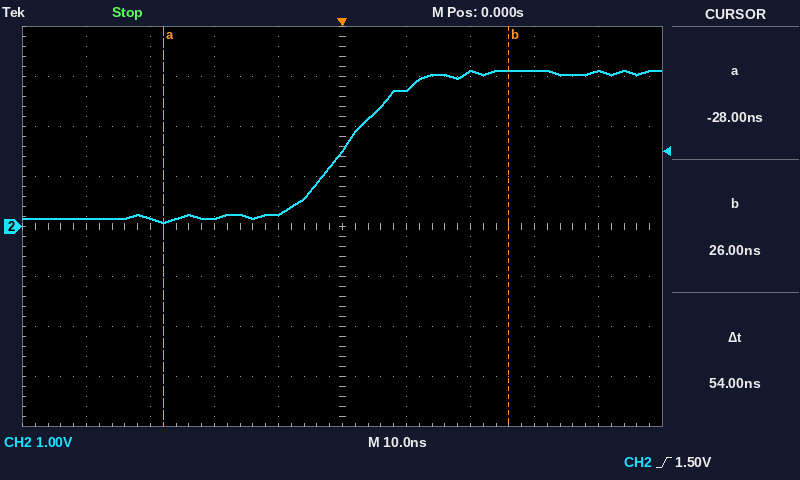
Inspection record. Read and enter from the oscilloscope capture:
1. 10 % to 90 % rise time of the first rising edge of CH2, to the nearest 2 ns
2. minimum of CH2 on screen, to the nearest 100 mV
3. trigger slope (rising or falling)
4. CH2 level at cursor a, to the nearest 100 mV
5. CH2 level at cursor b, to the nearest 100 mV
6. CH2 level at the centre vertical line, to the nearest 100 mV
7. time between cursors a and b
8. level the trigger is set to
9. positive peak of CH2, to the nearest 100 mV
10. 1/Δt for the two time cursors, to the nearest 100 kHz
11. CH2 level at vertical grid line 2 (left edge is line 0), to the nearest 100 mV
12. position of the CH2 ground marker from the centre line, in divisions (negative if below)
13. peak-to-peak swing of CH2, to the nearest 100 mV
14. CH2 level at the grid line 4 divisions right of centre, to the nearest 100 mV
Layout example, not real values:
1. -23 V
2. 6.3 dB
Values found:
1. 18 ns
2. 100 mV
3. rising
4. 100 mV
5. 3.1 V
6. 1.5 V
7. 54 ns
8. 1.50 V
9. 3.1 V
10. 18.5 MHz
11. 200 mV
12. 0.0 div
13. 3.0 V
14. 3.1 V
